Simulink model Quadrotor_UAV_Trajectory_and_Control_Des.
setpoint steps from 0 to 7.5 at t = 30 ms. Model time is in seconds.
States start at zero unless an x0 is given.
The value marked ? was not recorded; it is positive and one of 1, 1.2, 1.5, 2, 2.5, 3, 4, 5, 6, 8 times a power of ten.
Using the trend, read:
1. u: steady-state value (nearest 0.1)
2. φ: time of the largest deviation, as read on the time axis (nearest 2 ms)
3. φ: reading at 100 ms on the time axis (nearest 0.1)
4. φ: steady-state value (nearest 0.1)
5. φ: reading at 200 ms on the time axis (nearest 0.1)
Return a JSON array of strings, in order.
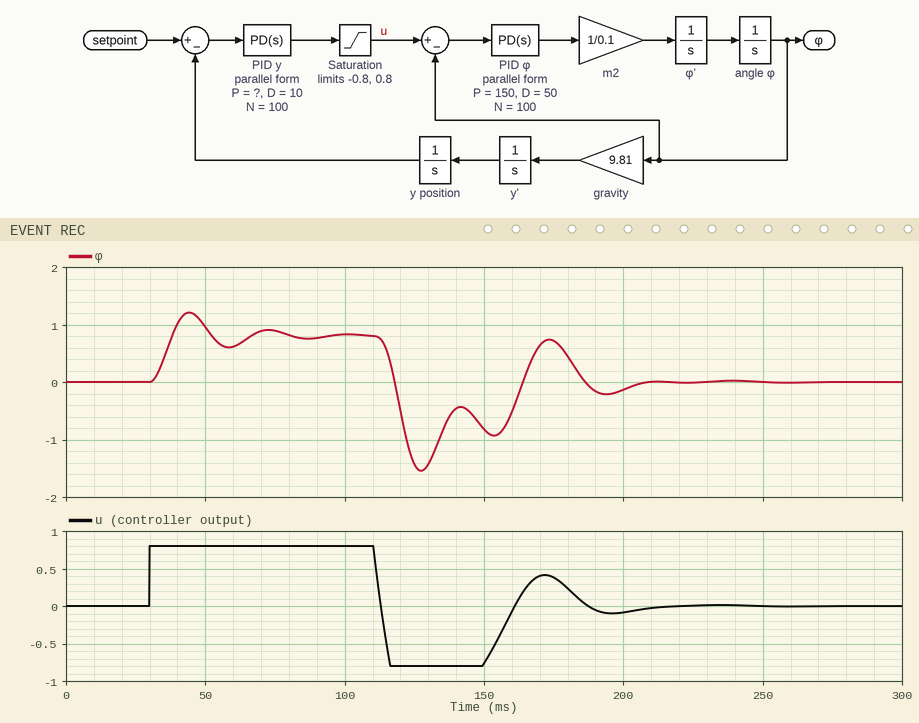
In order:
["0.0", "128 ms", "0.8", "0.0", "-0.1"]
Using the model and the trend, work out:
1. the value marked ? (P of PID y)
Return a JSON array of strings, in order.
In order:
["0.5"]
